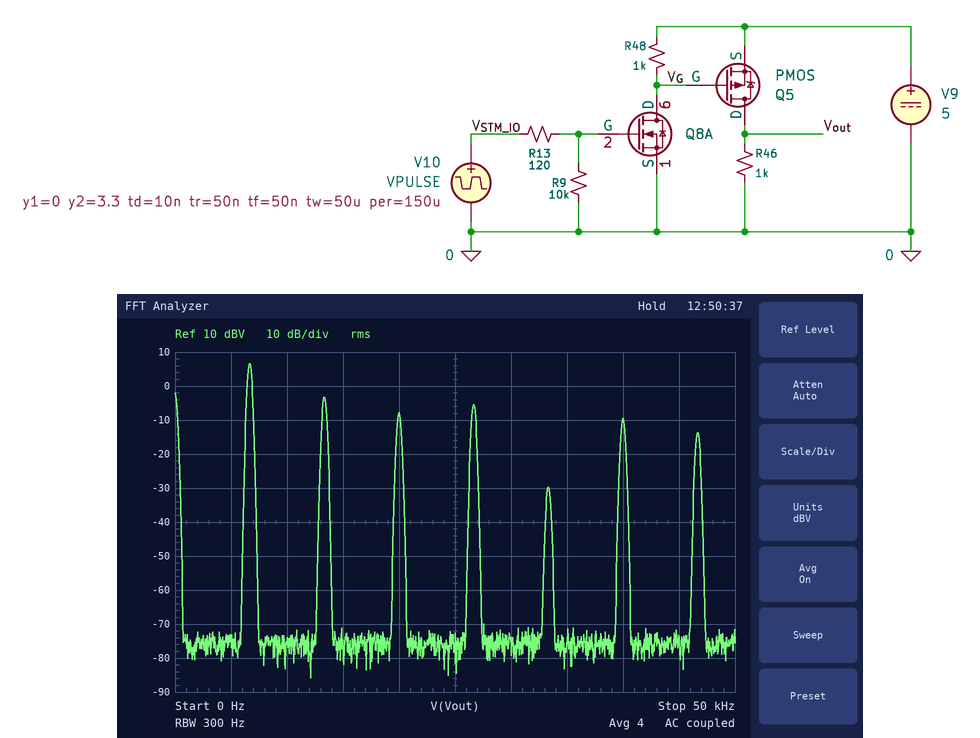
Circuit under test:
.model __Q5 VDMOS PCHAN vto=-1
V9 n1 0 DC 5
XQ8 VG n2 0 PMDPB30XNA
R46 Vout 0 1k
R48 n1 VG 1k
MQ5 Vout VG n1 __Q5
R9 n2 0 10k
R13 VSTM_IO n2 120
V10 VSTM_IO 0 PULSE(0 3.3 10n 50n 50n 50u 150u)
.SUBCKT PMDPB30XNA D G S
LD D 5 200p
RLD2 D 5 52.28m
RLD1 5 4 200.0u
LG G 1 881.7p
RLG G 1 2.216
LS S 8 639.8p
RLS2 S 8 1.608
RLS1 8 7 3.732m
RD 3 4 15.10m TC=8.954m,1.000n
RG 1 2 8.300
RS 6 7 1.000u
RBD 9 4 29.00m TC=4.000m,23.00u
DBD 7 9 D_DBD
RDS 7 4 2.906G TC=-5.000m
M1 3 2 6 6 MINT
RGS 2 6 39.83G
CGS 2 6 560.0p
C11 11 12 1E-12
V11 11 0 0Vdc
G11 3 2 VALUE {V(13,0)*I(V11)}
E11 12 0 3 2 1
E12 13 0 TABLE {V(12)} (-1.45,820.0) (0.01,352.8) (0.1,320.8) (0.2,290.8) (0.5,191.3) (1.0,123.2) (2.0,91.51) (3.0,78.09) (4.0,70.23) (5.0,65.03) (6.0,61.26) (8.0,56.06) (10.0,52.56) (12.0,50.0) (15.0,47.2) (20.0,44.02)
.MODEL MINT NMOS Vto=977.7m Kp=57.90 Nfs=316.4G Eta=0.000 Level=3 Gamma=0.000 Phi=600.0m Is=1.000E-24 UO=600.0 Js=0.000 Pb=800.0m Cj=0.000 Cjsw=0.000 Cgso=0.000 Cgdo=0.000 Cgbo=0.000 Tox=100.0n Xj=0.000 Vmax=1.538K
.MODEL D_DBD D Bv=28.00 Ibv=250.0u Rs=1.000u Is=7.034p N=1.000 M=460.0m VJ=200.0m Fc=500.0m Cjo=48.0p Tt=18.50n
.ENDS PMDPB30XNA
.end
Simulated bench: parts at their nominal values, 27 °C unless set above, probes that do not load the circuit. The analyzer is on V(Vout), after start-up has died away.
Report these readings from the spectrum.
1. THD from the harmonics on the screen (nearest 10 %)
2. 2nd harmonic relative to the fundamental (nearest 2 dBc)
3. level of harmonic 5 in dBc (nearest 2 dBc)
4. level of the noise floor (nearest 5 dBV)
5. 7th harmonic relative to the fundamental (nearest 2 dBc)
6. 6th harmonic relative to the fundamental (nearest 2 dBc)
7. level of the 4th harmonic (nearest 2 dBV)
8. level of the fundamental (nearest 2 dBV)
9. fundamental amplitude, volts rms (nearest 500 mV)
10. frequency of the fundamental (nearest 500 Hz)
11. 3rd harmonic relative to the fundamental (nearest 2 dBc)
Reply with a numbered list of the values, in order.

1. 50 %
2. -10 dBc
3. -36 dBc
4. -75 dBV
5. -20 dBc
6. -16 dBc
7. -6 dBV
8. 6 dBV
9. 2.0 V
10. 6.5 kHz
11. -14 dBc
